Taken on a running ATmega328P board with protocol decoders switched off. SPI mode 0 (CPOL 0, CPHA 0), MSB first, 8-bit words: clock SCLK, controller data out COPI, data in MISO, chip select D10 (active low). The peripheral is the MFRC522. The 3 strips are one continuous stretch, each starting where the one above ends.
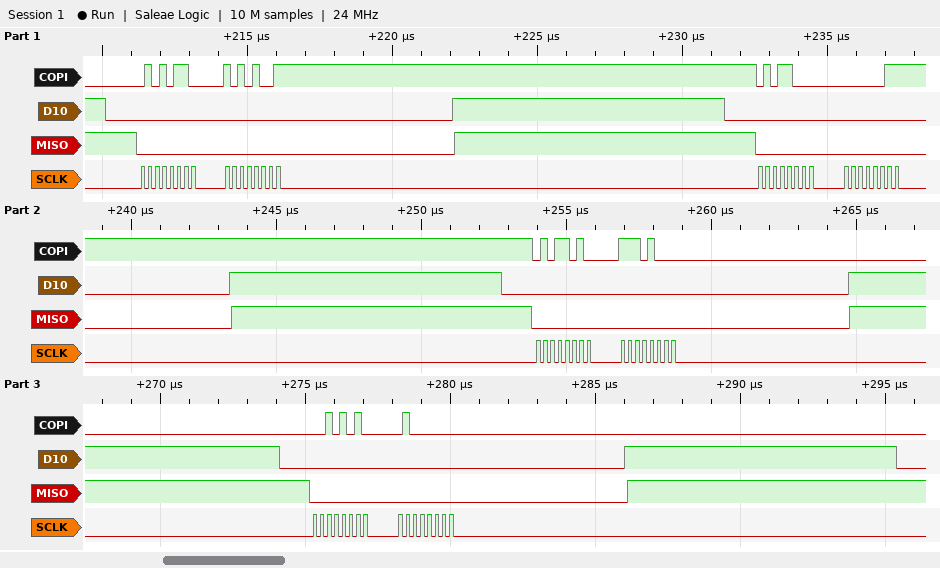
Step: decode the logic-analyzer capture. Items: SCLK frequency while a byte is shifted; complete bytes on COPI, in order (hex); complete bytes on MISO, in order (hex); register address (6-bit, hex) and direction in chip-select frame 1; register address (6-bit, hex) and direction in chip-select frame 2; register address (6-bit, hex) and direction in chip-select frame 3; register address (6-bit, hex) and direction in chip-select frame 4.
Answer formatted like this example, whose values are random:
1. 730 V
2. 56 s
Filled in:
1. 4 MHz
2. 0x56 0xA9 0x58 0x03 0x5A 0xE8 0x2A 0x40
3. 0x00 0x00 0x00 0x00 0x00 0x00 0x00 0x00
4. 0x2B write
5. 0x2C write
6. 0x2D write
7. 0x15 write
